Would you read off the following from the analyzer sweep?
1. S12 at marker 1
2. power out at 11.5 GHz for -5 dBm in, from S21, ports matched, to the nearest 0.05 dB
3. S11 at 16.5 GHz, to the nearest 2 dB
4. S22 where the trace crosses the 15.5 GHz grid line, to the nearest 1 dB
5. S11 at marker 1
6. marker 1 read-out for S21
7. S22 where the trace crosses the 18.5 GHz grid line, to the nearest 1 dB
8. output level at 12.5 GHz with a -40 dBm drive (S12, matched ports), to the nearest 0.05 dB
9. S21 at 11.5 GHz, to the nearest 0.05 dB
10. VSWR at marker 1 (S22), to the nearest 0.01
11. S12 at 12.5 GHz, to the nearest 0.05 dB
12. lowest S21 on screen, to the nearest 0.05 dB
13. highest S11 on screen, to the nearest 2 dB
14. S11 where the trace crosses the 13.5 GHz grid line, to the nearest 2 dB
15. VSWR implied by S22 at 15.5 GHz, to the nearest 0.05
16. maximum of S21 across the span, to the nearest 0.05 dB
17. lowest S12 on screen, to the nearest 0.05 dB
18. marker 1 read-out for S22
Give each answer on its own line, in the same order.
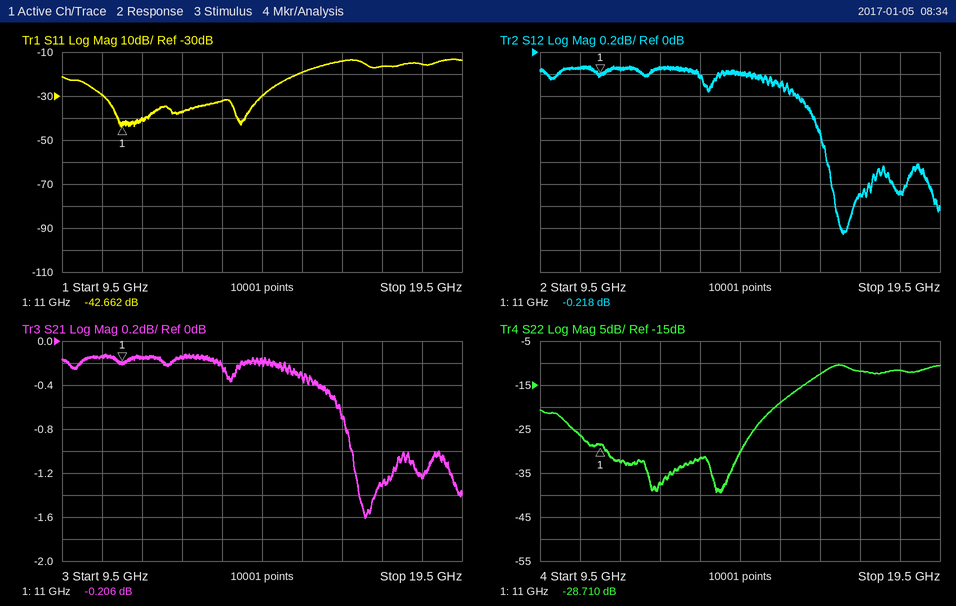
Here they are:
-0.218 dB
-5.15 dBm
-14 dB
-19 dB
-42.662 dB
-0.206 dB
-12 dB
-40.15 dBm
-0.15 dB
1.08
-0.15 dB
-1.60 dB
-14 dB
-32 dB
1.25
-0.10 dB
-1.65 dB
-28.710 dB
